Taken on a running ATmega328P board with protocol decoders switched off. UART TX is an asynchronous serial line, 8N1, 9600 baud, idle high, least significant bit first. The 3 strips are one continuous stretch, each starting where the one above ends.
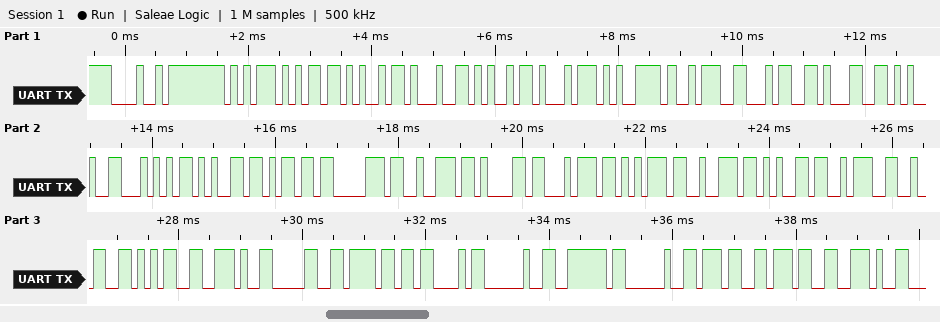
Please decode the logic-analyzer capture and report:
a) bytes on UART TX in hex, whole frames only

48 75 6D 69 64 69 74 79 3A 34 31 25 54 65 6D 70 72 61 74 75 72 65 3A 32 35 2E 30 6F 43 20 7E 20 37 37 2E
